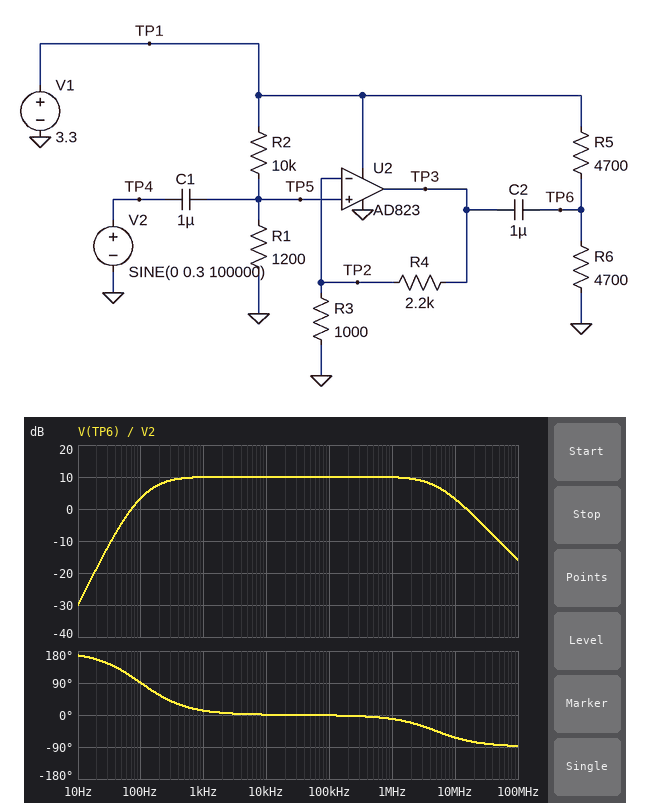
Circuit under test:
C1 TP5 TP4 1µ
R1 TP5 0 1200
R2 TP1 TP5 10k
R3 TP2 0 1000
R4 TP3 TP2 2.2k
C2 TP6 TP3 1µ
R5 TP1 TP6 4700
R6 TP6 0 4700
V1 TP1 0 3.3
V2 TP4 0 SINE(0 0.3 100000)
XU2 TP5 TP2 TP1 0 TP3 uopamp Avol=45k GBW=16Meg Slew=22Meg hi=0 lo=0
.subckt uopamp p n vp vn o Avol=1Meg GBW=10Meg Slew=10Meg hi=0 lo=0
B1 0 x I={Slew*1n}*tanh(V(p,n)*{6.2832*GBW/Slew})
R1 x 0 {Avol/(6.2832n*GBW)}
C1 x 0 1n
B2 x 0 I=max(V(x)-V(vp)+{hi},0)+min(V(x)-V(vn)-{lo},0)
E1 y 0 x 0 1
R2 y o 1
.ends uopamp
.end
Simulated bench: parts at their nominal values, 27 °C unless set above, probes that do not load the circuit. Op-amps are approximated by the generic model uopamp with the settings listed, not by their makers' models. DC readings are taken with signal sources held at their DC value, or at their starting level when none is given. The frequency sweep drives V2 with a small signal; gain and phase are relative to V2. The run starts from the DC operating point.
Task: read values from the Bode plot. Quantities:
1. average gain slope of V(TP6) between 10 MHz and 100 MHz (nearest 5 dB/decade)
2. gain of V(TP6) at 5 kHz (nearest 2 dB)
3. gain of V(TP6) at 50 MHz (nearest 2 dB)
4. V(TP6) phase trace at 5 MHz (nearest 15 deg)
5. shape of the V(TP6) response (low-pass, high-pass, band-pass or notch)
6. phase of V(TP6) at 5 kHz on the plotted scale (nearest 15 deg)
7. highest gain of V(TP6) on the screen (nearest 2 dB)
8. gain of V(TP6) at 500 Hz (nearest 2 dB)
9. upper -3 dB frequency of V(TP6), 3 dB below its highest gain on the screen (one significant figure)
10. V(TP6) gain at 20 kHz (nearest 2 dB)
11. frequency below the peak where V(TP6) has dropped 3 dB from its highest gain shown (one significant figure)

-20 dB/decade
10 dB
-10 dB
-45 deg
band-pass
0 deg
10 dB
10 dB
5 MHz
10 dB
200 Hz
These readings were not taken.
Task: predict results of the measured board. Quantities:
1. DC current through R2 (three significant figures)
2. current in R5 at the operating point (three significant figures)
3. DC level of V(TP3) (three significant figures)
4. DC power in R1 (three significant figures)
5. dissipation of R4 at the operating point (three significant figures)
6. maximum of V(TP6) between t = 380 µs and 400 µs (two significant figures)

295 µA
351 µA
1.13 V
104 µW
275 µW
2.6 V
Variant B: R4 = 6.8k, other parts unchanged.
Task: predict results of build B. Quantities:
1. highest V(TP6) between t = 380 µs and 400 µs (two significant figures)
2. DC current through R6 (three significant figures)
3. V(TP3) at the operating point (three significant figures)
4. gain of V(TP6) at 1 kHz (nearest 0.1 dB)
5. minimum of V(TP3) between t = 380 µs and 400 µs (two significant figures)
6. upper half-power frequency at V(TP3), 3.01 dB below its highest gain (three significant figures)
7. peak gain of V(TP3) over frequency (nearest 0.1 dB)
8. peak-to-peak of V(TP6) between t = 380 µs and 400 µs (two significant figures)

2.3 V
351 µA
2.76 V
17.7 dB
420 mV
2.05 MHz
17.8 dB
2.9 V
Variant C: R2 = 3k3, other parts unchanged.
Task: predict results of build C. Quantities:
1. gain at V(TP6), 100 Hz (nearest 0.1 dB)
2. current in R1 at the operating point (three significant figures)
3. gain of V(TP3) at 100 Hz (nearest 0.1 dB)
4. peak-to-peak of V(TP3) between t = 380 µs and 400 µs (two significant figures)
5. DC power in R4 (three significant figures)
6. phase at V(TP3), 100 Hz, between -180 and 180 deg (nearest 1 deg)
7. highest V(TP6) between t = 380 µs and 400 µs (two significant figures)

2.2 dB
733 µA
3.8 dB
1.5 V
1.70 mW
61 deg
2.2 V
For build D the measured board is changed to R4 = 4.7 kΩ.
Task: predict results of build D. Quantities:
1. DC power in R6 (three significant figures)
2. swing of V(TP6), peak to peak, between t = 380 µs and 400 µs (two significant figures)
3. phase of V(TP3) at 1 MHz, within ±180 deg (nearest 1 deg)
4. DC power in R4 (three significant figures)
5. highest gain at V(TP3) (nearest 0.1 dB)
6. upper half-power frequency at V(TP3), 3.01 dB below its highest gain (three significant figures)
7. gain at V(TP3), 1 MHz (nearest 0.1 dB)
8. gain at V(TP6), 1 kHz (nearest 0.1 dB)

579 µW
3.0 V
-20 deg
587 µW
15.1 dB
2.81 MHz
14.6 dB
15.0 dB
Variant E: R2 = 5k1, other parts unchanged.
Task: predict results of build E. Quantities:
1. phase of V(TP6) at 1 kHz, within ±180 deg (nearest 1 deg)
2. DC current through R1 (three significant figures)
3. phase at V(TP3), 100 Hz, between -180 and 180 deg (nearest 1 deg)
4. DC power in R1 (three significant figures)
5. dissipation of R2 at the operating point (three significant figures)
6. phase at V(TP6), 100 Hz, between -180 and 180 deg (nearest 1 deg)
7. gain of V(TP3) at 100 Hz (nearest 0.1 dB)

13 deg
524 µA
59 deg
329 µW
1.40 mW
93 deg
4.4 dB
